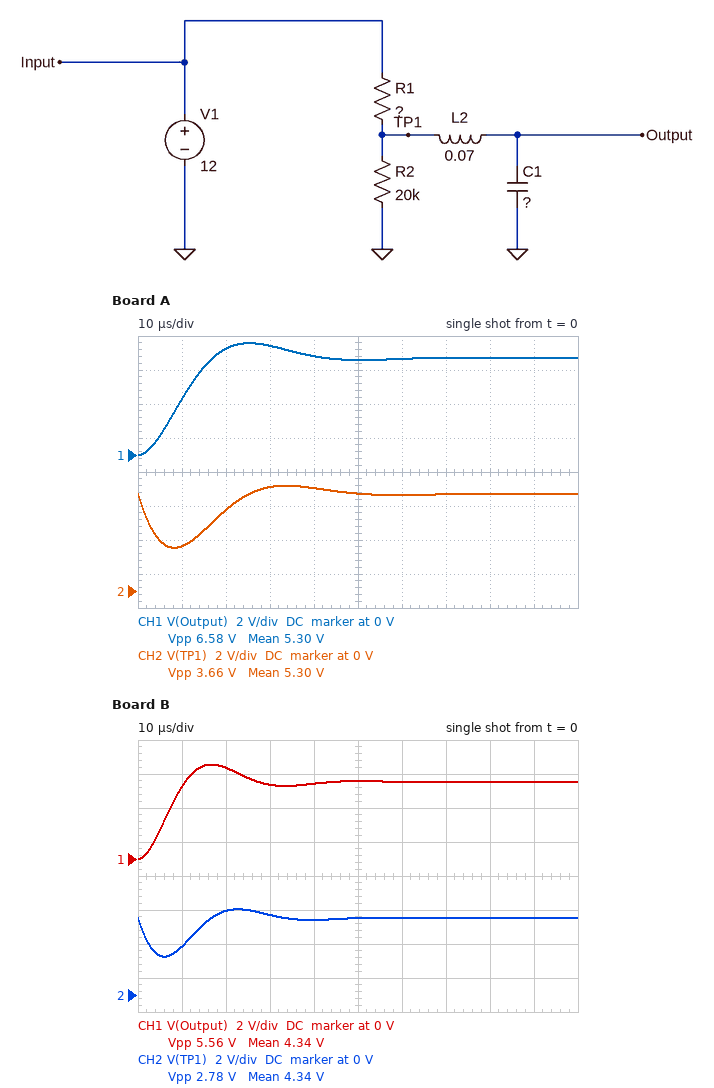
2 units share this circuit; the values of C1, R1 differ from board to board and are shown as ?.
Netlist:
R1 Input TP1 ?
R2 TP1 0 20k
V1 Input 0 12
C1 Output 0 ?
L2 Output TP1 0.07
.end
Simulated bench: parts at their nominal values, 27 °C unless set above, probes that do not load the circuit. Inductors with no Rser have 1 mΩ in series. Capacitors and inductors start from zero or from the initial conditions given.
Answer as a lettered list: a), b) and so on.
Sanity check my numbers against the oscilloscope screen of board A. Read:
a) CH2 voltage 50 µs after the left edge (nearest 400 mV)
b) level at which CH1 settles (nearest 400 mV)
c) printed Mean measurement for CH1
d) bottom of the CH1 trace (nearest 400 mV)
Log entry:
a) 5.6 V
b) 5.6 V
c) 5.30 V
d) 0 V
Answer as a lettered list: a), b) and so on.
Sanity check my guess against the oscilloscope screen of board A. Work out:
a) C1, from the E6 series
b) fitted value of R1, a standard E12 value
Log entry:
a) 680 pF
b) 22 kΩ
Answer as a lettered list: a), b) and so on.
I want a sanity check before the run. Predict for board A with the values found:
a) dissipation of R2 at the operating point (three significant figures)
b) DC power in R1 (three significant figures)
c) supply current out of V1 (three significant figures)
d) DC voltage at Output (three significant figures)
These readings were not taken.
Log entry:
a) 1.63 mW
b) 1.80 mW
c) 286 µA
d) 5.71 V
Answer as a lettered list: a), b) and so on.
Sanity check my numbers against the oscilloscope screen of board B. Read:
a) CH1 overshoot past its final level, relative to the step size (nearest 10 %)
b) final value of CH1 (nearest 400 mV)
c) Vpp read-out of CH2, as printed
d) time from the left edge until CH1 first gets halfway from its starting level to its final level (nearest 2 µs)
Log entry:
a) 20 %
b) 4.4 V
c) 2.78 V
d) 6 µs
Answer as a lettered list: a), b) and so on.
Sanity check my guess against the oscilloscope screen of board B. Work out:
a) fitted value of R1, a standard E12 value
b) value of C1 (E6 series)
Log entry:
a) 33 kΩ
b) 330 pF
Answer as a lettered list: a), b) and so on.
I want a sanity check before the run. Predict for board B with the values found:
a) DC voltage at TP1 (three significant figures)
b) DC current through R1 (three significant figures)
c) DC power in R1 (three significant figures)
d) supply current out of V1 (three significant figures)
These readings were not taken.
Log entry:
a) 4.53 V
b) 226 µA
c) 1.69 mW
d) 226 µA
